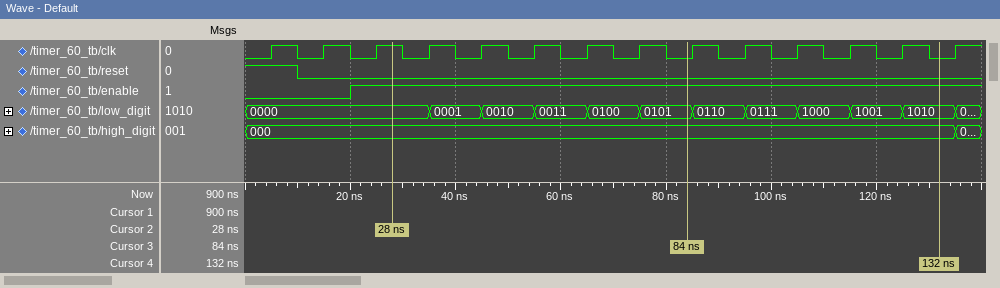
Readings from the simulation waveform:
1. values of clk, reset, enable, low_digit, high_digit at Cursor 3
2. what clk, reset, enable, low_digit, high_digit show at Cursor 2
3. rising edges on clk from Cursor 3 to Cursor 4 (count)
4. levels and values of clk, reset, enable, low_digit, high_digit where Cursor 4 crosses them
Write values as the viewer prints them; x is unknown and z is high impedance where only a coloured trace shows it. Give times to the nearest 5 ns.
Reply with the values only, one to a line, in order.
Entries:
clk=0, reset=0, enable=1, low_digit=0101, high_digit=000
clk=1, reset=0, enable=1, low_digit=0000, high_digit=000
5
clk=0, reset=0, enable=1, low_digit=1010, high_digit=000
